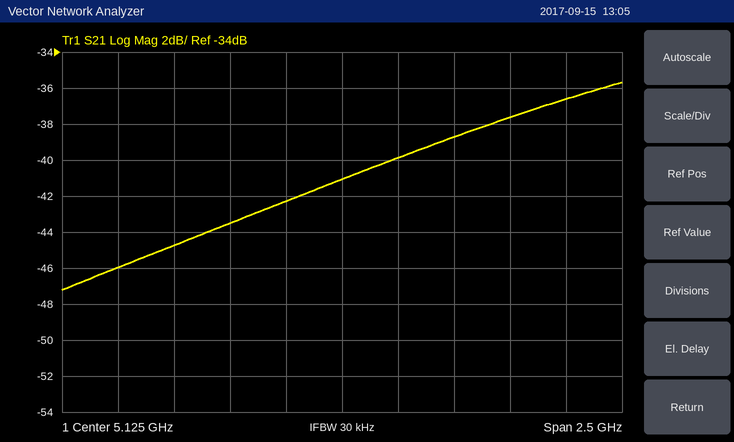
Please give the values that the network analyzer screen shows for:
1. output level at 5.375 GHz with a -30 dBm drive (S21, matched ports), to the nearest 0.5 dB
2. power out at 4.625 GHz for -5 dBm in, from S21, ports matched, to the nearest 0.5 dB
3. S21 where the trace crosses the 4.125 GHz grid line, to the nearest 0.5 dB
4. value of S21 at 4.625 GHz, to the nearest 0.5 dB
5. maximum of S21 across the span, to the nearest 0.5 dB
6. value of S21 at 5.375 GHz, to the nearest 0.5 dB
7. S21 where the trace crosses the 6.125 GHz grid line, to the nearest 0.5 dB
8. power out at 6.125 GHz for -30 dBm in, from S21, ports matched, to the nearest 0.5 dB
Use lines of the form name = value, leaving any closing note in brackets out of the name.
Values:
output level at 5.375 GHz with a -30 dBm drive (S21, matched ports), to the nearest 0.5 dB = -70.0 dBm
power out at 4.625 GHz for -5 dBm in, from S21, ports matched, to the nearest 0.5 dB = -48.5 dBm
S21 where the trace crosses the 4.125 GHz grid line, to the nearest 0.5 dB = -46.0 dB
value of S21 at 4.625 GHz, to the nearest 0.5 dB = -43.5 dB
maximum of S21 across the span, to the nearest 0.5 dB = -35.5 dB
value of S21 at 5.375 GHz, to the nearest 0.5 dB = -40.0 dB
S21 where the trace crosses the 6.125 GHz grid line, to the nearest 0.5 dB = -36.5 dB
power out at 6.125 GHz for -30 dBm in, from S21, ports matched, to the nearest 0.5 dB = -66.5 dBm
